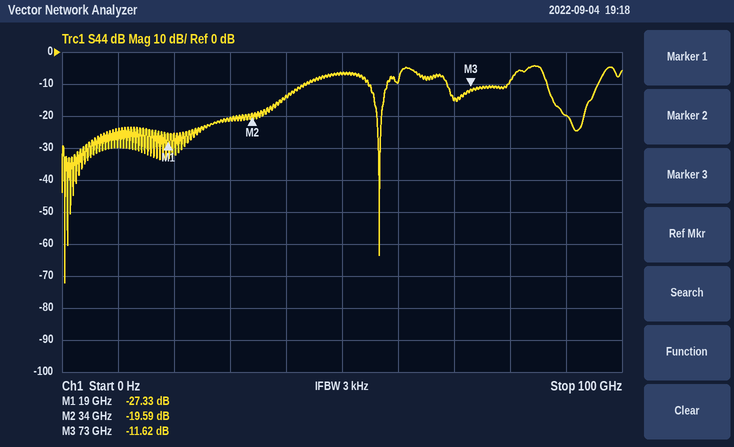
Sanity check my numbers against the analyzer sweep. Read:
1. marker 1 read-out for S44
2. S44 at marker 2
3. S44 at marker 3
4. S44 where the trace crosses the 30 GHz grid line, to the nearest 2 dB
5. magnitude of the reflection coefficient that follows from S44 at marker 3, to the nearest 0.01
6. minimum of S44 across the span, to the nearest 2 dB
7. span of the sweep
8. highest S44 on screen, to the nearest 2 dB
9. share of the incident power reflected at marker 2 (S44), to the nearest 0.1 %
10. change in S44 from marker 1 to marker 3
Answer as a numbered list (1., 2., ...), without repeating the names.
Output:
1. -27.33 dB
2. -19.59 dB
3. -11.62 dB
4. -20 dB
5. 0.26
6. -72 dB
7. 100 GHz
8. -4 dB
9. 1.1 %
10. 15.71 dB
